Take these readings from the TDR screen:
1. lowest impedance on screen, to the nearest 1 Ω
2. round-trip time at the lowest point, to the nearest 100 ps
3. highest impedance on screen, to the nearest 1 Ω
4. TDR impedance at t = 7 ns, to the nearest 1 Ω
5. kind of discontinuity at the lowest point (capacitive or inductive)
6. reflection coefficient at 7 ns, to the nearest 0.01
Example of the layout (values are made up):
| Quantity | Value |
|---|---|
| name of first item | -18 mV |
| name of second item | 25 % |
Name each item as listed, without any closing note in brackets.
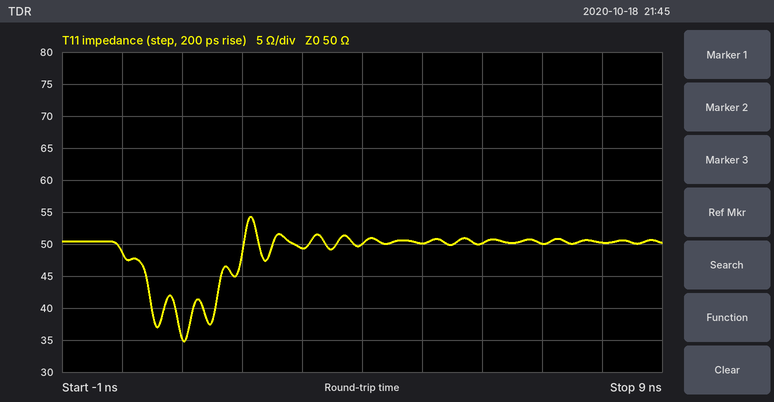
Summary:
| Quantity | Value |
|---|---|
| lowest impedance on screen, to the nearest 1 Ω | 35 Ω |
| round-trip time at the lowest point, to the nearest 100 ps | 1.0 ns |
| highest impedance on screen, to the nearest 1 Ω | 54 Ω |
| TDR impedance at t = 7 ns, to the nearest 1 Ω | 50 Ω |
| kind of discontinuity at the lowest point | capacitive |
| reflection coefficient at 7 ns, to the nearest 0.01 | 0.00 |
